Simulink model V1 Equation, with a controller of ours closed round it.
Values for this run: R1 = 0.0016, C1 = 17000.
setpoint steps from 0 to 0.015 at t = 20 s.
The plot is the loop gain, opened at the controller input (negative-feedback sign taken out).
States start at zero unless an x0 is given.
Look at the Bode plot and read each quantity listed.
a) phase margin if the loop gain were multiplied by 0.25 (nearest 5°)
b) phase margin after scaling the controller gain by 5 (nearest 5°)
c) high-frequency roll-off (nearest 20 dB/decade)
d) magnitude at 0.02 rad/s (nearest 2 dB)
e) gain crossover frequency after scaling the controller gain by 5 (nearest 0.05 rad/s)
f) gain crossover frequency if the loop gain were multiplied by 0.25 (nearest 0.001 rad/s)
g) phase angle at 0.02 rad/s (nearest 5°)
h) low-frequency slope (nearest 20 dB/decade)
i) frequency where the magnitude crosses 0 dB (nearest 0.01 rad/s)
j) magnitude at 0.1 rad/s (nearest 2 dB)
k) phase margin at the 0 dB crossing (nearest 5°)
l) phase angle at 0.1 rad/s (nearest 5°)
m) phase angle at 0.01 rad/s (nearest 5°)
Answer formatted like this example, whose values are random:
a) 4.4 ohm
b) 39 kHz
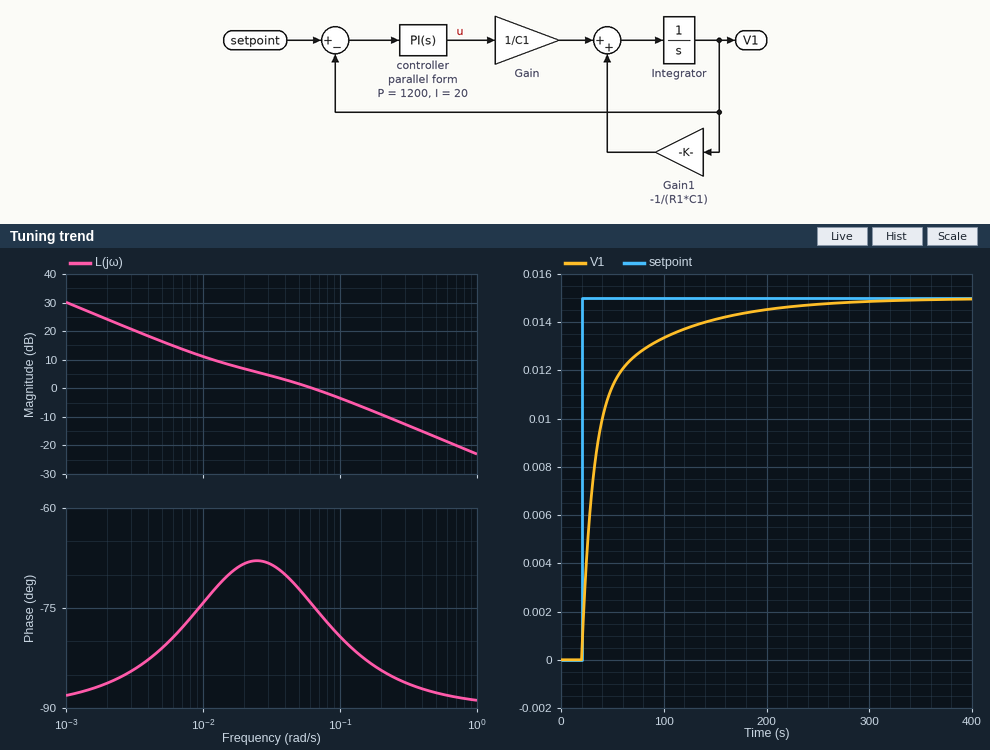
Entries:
a) 105°
b) 95°
c) -20 dB/decade
d) 6 dB
e) 0.35 rad/s
f) 0.009 rad/s
g) -70°
h) -20 dB/decade
i) 0.06 rad/s
j) -4 dB
k) 105°
l) -80°
m) -75°
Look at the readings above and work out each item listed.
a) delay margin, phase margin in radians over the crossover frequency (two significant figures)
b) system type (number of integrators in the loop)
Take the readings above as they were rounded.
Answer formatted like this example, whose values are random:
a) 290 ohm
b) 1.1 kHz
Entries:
a) 31 s
b) 1
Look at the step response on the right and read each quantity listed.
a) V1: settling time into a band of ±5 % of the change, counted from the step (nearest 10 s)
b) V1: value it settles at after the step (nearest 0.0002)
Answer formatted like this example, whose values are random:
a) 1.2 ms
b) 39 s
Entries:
a) 140 s
b) 0.0150
